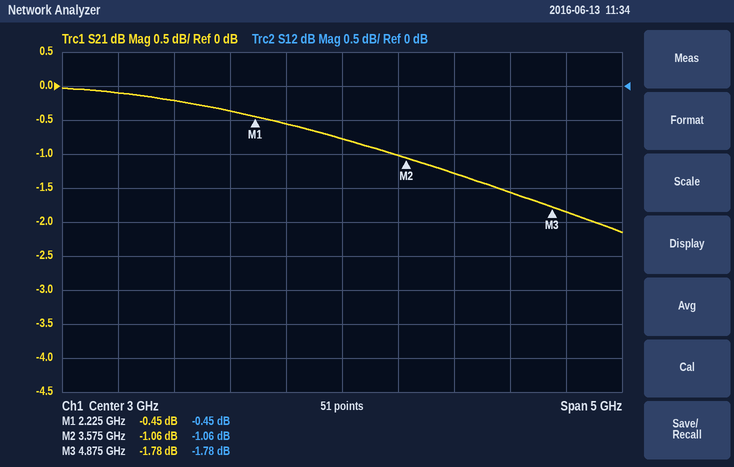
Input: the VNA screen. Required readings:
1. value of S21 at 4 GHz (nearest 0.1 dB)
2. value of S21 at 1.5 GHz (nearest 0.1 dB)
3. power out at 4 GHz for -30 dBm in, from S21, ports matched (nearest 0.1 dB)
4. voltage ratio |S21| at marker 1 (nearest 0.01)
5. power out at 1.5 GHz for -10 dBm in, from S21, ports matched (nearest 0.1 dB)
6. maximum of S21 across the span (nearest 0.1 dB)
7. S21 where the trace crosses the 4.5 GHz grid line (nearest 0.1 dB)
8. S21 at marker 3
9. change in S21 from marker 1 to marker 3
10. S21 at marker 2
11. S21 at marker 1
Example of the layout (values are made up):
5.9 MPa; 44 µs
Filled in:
-1.3 dB; -0.2 dB; -31.3 dBm; 0.95; -10.2 dBm; 0.0 dB; -1.6 dB; -1.78 dB; -1.33 dB; -1.06 dB; -0.45 dB
